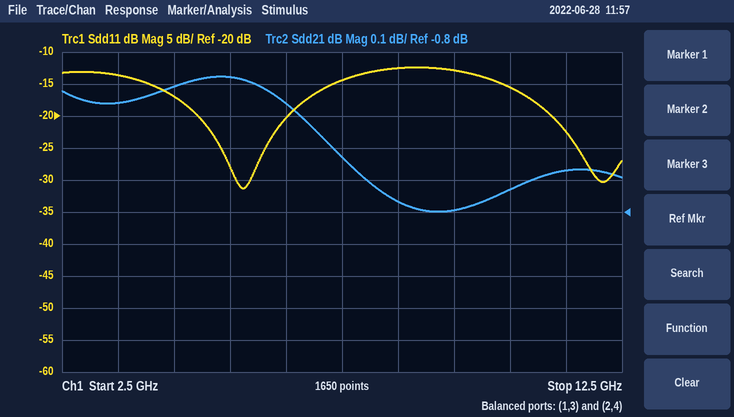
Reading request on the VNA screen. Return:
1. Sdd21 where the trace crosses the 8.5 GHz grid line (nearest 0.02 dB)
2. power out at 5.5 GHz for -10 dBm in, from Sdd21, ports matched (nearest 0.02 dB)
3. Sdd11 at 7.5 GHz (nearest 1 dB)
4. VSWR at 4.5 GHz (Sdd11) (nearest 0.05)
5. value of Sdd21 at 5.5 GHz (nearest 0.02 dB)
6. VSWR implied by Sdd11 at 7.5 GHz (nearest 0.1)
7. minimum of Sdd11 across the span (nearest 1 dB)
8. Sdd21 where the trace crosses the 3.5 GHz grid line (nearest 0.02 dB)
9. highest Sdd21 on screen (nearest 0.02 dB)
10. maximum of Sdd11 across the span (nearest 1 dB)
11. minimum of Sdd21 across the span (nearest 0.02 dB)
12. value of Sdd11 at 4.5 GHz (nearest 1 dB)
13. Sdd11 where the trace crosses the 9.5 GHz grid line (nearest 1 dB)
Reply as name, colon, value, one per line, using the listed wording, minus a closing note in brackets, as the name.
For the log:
Sdd21 where the trace crosses the 8.5 GHz grid line: -0.76 dB
power out at 5.5 GHz for -10 dBm in, from Sdd21, ports matched: -10.38 dBm
Sdd11 at 7.5 GHz: -14 dB
VSWR at 4.5 GHz (Sdd11): 1.35
value of Sdd21 at 5.5 GHz: -0.38 dB
VSWR implied by Sdd11 at 7.5 GHz: 1.5
minimum of Sdd11 across the span: -31 dB
Sdd21 where the trace crosses the 3.5 GHz grid line: -0.46 dB
highest Sdd21 on screen: -0.38 dB
maximum of Sdd11 across the span: -12 dB
minimum of Sdd21 across the span: -0.80 dB
value of Sdd11 at 4.5 GHz: -17 dB
Sdd11 where the trace crosses the 9.5 GHz grid line: -13 dB
